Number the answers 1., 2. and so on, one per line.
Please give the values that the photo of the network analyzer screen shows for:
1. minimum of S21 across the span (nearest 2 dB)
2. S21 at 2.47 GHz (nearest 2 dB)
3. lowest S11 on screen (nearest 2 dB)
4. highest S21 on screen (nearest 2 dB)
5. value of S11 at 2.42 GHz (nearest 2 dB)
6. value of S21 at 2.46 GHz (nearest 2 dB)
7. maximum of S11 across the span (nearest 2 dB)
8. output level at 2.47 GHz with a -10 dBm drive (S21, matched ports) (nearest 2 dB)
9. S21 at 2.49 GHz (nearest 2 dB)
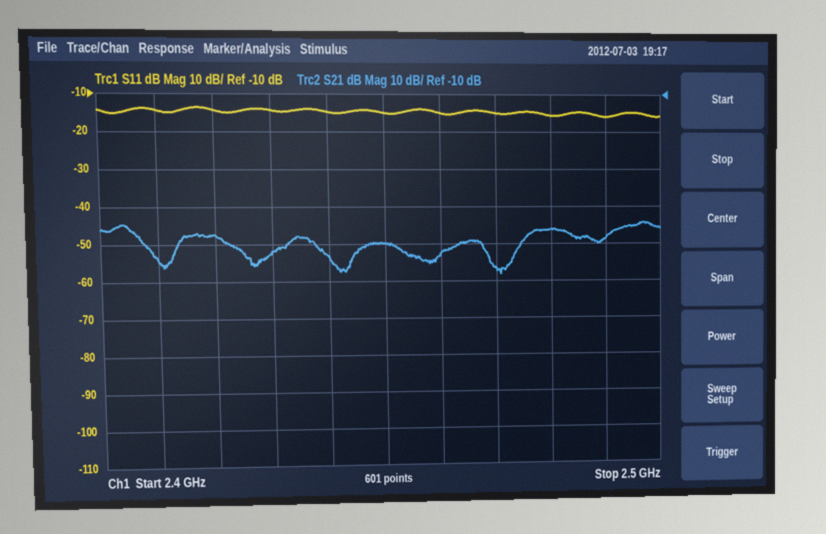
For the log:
1. -58 dB
2. -56 dB
3. -16 dB
4. -44 dB
5. -14 dB
6. -52 dB
7. -14 dB
8. -66 dBm
9. -48 dB
